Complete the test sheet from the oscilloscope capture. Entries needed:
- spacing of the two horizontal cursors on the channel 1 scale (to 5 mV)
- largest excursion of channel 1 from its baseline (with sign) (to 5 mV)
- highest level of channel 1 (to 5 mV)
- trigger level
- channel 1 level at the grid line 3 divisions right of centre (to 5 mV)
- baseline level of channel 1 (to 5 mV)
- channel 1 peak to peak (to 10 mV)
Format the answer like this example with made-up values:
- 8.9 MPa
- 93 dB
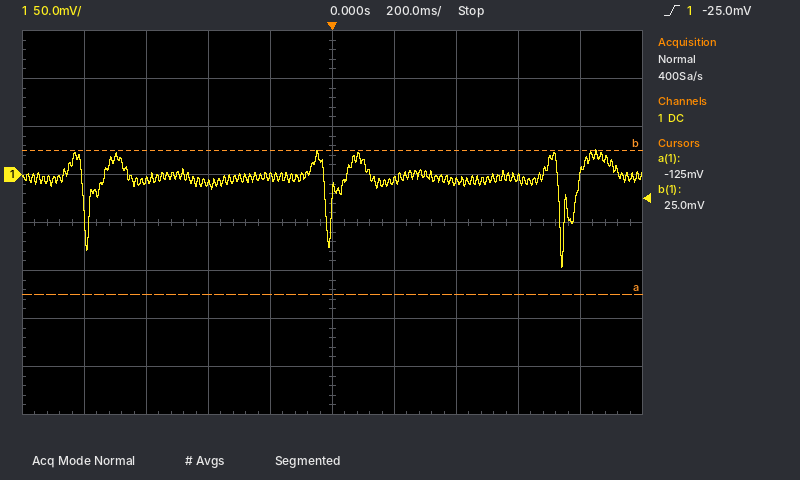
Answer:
- 150 mV
- -95 mV
- 25 mV
- -25.0 mV
- -5 mV
- -5 mV
- 120 mV
